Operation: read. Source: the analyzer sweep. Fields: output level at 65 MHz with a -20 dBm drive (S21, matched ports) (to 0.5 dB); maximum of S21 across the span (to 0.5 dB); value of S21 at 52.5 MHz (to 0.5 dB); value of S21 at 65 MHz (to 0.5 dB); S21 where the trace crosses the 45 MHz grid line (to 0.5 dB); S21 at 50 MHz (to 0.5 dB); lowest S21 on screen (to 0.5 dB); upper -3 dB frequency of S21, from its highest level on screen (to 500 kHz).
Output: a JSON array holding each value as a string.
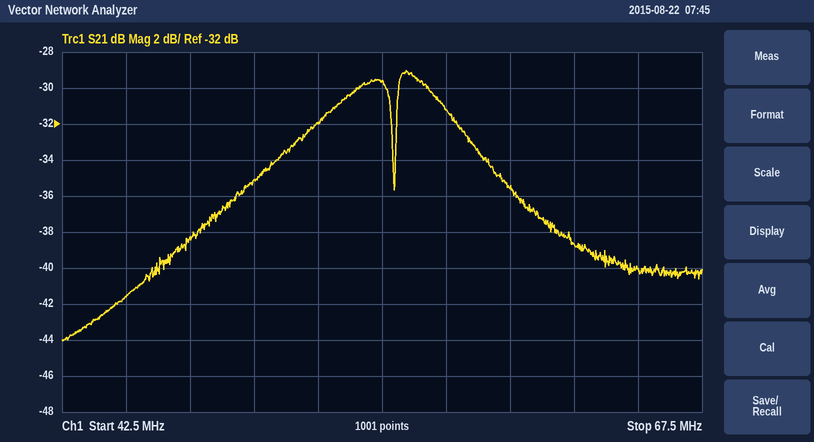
["-60.0 dBm", "-29.0 dB", "-32.0 dB", "-40.0 dB", "-41.5 dB", "-35.0 dB", "-44.0 dB", "58.0 MHz"]
